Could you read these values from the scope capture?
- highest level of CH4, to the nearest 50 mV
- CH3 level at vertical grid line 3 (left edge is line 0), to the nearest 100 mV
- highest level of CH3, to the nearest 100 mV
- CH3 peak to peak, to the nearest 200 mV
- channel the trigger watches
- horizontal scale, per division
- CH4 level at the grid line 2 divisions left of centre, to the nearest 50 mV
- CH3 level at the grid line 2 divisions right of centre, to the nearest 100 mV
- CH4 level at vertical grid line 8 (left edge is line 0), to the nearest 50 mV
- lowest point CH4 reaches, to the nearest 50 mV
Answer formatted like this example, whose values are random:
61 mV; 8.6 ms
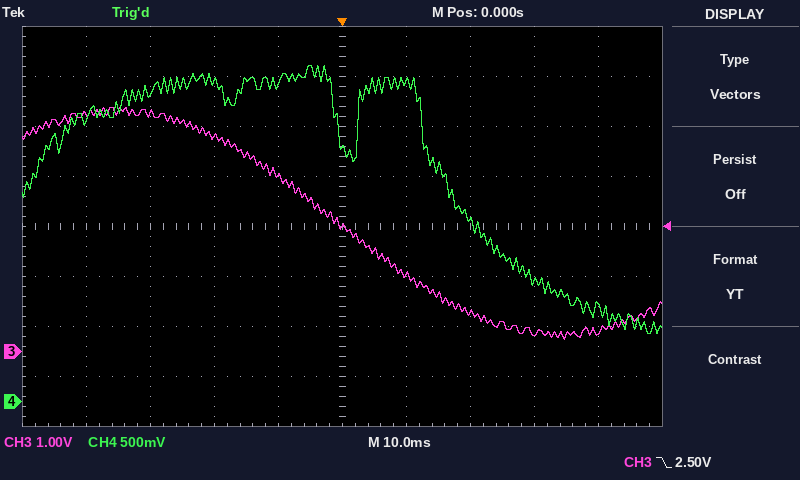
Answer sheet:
3.35 V; 4.3 V; 4.9 V; 4.6 V; CH3; 10 ms; 3.20 V; 800 mV; 1.20 V; 700 mV
